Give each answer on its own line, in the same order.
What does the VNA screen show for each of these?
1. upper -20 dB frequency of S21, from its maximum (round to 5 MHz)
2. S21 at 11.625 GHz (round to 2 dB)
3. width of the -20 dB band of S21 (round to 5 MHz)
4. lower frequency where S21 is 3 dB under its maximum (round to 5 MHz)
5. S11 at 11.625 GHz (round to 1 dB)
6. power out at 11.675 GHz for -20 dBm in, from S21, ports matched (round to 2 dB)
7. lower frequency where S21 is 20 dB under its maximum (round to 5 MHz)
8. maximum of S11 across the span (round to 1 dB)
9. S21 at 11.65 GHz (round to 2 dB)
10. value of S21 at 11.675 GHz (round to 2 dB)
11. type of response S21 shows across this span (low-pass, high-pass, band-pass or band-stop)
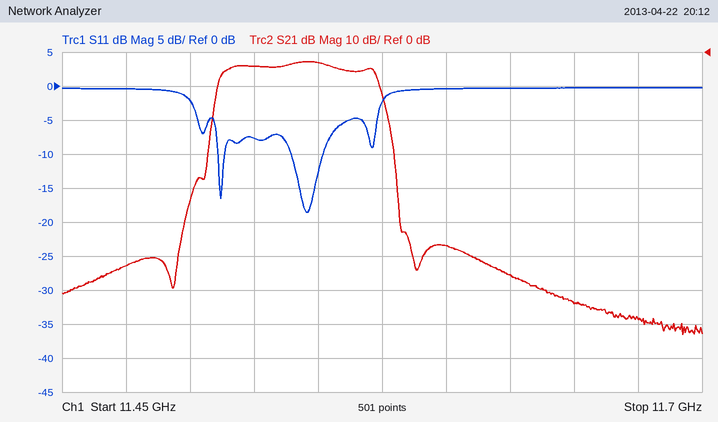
11.580 GHz
-66 dB
70 MHz
11.515 GHz
0 dB
-98 dBm
11.510 GHz
0 dB
-74 dB
-78 dB
band-pass
